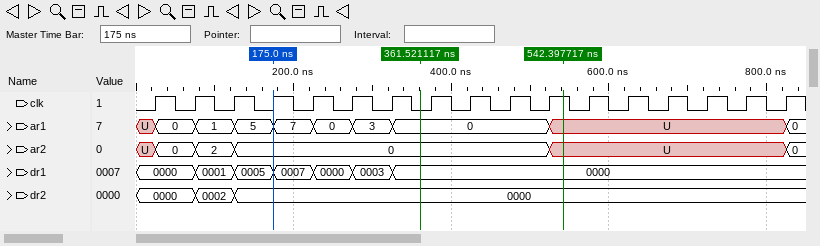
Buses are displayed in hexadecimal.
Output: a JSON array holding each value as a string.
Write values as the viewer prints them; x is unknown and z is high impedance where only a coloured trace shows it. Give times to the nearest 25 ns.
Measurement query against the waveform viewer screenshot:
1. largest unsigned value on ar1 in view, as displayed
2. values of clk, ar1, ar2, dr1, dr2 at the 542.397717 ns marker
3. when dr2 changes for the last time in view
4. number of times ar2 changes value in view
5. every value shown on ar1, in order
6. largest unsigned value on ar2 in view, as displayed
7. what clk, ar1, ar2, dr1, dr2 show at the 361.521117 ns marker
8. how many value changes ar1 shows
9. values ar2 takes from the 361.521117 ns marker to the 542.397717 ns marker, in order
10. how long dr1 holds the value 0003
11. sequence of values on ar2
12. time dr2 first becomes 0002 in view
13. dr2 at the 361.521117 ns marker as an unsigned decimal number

["7", "clk=1, ar1=U, ar2=U, dr1=0000, dr2=0000", "125 ns", "5", "U, 0, 1, 5, 7, 0, 3, 0, U, 0", "2", "clk=0, ar1=0, ar2=0, dr1=0000, dr2=0000", "9", "0, U", "50 ns", "U, 0, 2, 0, U, 0", "75 ns", "0"]
